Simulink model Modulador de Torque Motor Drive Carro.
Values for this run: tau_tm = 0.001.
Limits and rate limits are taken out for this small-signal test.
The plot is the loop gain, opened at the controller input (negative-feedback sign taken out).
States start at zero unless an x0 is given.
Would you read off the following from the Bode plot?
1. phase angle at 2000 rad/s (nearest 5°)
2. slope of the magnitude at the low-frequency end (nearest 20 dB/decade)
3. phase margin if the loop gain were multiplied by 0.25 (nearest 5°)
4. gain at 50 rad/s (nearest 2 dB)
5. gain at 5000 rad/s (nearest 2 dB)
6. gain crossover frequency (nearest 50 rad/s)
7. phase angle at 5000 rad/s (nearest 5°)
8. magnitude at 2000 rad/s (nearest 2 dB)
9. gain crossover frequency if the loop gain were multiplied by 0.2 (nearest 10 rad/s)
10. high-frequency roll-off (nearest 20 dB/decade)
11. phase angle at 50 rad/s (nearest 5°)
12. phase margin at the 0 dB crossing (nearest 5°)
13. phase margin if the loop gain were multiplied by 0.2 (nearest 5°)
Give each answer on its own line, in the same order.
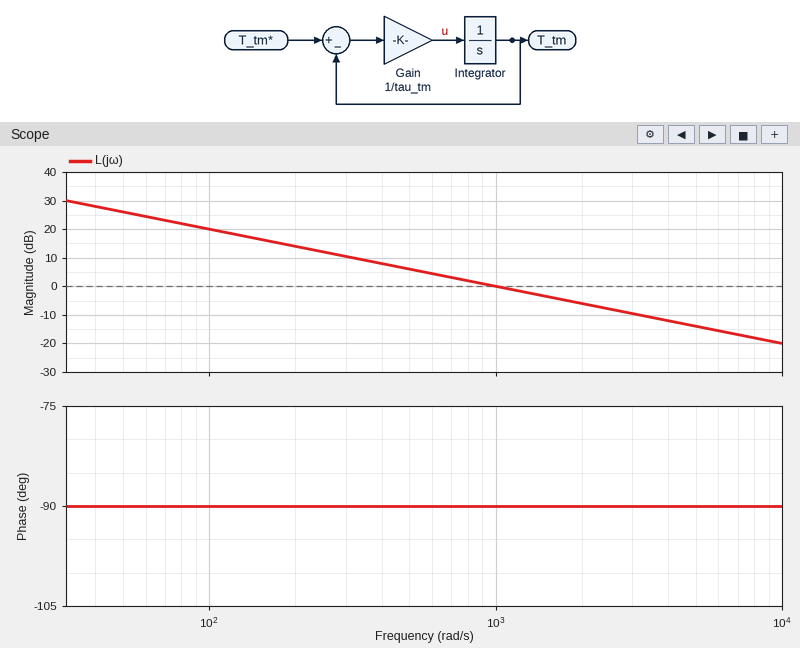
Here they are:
-90°
-20 dB/decade
90°
26 dB
-14 dB
1000 rad/s
-90°
-6 dB
200 rad/s
-20 dB/decade
-90°
90°
90°
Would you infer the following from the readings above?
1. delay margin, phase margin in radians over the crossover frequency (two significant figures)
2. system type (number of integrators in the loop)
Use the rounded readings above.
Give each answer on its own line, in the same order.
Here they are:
0.0016 s
1
